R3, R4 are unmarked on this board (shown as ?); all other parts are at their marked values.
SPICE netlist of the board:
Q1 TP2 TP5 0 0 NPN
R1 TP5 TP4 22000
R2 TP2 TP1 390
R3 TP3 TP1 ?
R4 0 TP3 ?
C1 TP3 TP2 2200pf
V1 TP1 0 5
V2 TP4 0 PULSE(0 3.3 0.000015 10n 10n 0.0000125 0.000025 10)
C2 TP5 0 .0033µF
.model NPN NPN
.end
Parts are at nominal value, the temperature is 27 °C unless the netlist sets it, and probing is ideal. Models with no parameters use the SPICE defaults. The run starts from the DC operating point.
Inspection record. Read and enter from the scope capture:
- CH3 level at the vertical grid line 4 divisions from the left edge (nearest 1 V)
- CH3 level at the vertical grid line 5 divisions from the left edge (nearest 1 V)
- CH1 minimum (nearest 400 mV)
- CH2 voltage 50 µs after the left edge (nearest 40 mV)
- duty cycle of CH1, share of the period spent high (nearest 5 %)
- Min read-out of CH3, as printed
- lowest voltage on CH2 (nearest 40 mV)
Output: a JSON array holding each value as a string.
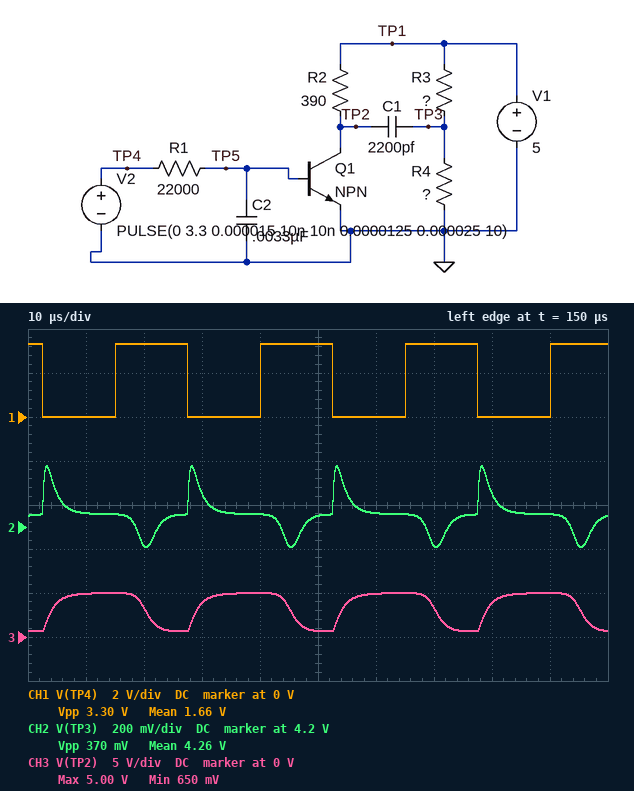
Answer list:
["5 V", "1 V", "0 V", "4.24 V", "50 %", "650 mV", "4.12 V"]
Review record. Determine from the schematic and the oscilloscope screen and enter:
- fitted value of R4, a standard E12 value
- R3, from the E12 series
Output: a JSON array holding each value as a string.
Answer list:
["390 Ω", "68 Ω"]
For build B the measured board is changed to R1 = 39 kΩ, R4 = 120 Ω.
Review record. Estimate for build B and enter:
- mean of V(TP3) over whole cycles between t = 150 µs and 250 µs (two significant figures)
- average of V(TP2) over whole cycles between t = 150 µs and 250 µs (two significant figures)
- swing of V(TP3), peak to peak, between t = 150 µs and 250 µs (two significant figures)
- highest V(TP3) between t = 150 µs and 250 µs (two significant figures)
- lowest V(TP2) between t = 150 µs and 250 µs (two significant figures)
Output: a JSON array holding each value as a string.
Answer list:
["3.2 V", "4.1 V", "110 mV", "3.3 V", "2.6 V"]
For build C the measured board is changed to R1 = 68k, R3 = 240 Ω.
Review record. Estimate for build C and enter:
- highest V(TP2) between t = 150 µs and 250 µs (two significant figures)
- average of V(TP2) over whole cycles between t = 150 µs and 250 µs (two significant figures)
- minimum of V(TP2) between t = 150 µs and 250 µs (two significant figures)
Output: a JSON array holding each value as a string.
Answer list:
["4.9 V", "4.5 V", "3.7 V"]
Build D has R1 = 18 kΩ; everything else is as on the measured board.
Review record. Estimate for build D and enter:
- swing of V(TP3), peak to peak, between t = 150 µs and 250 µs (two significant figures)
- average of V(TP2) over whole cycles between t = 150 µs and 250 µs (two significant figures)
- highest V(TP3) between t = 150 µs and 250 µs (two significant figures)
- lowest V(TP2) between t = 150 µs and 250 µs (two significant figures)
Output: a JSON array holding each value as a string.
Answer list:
["470 mV", "3.2 V", "4.5 V", "160 mV"]
